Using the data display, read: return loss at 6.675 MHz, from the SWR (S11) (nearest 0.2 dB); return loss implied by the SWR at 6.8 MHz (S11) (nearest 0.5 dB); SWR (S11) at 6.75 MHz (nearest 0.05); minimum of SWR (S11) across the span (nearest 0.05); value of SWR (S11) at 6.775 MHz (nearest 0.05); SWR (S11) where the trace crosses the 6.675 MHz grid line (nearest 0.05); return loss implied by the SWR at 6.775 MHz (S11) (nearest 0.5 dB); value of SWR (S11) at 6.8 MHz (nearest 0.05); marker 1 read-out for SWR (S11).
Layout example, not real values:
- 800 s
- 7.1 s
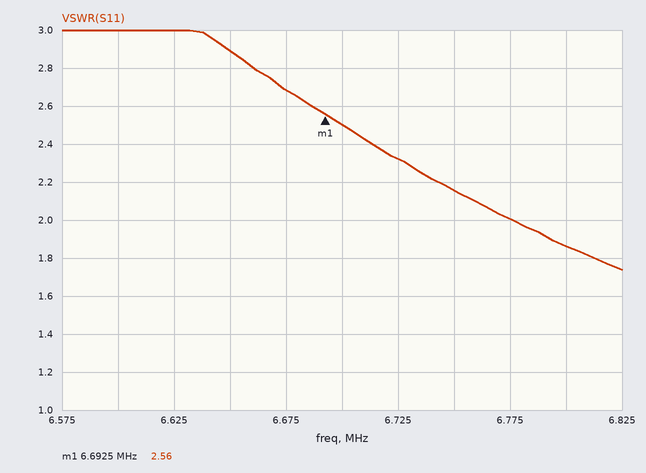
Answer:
- 6.8 dB
- 10.5 dB
- 2.15
- 1.75
- 2.00
- 2.70
- 9.5 dB
- 1.85
- 2.56
